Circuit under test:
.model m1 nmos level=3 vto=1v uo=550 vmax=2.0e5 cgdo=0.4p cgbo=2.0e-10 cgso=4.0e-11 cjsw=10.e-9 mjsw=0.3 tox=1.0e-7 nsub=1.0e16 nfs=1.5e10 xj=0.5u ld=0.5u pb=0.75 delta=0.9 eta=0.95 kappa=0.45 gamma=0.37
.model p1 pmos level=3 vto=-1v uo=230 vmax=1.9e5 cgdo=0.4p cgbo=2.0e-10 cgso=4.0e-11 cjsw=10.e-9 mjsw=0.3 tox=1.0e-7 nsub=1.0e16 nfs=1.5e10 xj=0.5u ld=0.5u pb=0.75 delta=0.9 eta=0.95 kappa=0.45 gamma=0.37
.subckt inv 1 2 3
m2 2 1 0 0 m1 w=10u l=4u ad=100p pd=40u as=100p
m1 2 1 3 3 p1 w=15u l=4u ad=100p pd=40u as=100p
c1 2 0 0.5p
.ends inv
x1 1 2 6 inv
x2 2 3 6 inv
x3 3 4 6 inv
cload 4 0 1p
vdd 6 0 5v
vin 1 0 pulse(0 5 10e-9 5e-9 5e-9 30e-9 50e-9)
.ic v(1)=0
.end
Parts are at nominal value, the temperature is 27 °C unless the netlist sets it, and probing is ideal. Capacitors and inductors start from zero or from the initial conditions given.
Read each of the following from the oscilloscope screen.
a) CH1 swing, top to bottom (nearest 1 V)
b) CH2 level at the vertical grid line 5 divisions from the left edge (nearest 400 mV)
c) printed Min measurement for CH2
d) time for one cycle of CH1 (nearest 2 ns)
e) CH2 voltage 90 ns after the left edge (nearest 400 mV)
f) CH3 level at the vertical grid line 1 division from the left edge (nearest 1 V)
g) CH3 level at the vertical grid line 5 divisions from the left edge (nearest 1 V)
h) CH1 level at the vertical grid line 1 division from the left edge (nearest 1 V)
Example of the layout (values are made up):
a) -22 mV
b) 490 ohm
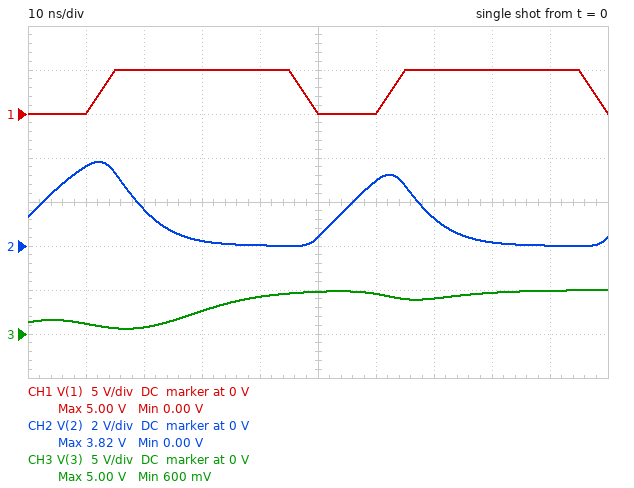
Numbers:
a) 5 V
b) 400 mV
c) 0.00 V
d) 50 ns
e) 0 V
f) 1 V
g) 5 V
h) 0 V
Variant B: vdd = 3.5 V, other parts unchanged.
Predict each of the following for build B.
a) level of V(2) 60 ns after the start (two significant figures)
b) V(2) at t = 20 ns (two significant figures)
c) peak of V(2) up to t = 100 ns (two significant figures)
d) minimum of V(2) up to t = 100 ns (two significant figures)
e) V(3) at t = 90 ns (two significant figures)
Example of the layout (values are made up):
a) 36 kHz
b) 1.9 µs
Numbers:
a) 1.2 V
b) 650 mV
c) 2.1 V
d) -8.5 mV
e) 3.5 V
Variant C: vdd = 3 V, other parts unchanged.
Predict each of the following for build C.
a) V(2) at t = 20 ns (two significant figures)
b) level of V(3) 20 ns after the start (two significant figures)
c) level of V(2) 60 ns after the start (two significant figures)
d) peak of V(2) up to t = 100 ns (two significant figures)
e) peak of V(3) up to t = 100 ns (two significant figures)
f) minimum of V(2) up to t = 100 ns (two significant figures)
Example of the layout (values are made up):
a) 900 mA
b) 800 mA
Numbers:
a) 450 mV
b) 1.1 V
c) 750 mV
d) 1.6 V
e) 3.0 V
f) -11 mV
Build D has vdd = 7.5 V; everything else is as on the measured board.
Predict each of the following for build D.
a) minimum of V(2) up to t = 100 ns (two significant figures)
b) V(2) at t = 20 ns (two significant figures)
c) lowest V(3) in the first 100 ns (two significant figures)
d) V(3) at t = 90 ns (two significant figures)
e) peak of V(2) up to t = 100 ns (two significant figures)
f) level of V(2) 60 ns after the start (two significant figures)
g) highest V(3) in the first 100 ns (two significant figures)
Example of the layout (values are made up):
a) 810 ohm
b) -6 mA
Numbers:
a) 380 mV
b) 4.5 V
c) 110 mV
d) 6.4 V
e) 6.9 V
f) 6.6 V
g) 7.3 V
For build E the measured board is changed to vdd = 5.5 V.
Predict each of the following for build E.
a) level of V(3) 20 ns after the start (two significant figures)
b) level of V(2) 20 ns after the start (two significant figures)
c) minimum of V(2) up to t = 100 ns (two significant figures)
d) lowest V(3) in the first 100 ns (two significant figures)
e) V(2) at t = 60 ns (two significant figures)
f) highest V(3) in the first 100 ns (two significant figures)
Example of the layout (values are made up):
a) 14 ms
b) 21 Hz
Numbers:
a) 560 mV
b) 2.1 V
c) 7.1 mV
d) 440 mV
e) 3.7 V
f) 5.5 V
